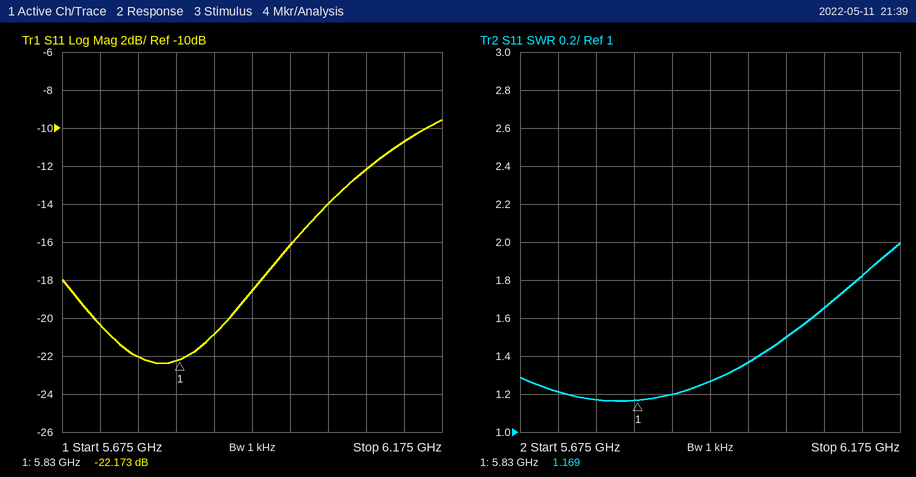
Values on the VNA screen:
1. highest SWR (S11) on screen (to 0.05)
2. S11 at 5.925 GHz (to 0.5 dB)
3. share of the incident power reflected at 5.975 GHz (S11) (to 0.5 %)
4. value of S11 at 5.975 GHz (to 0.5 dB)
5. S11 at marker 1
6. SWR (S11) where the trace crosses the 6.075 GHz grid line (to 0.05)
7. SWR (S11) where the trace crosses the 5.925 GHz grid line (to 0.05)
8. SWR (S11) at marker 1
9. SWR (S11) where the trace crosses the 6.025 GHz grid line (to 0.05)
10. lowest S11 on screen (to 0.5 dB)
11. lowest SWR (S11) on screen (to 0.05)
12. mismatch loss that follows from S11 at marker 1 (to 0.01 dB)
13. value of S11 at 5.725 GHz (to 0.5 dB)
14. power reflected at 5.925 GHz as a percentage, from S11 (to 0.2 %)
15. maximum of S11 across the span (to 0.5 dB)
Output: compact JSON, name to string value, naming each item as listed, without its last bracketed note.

{"highest SWR (S11) on screen": "2.00", "S11 at 5.925 GHz": "-18.5 dB", "share of the incident power reflected at 5.975 GHz (S11)": "2.5 %", "value of S11 at 5.975 GHz": "-16.0 dB", "S11 at marker 1": "-22.173 dB", "SWR (S11) where the trace crosses the 6.075 GHz grid line": "1.65", "SWR (S11) where the trace crosses the 5.925 GHz grid line": "1.25", "SWR (S11) at marker 1": "1.169", "SWR (S11) where the trace crosses the 6.025 GHz grid line": "1.50", "lowest S11 on screen": "-22.5 dB", "lowest SWR (S11) on screen": "1.15", "mismatch loss that follows from S11 at marker 1": "0.03 dB", "value of S11 at 5.725 GHz": "-20.5 dB", "power reflected at 5.925 GHz as a percentage, from S11": "1.4 %", "maximum of S11 across the span": "-9.5 dB"}
